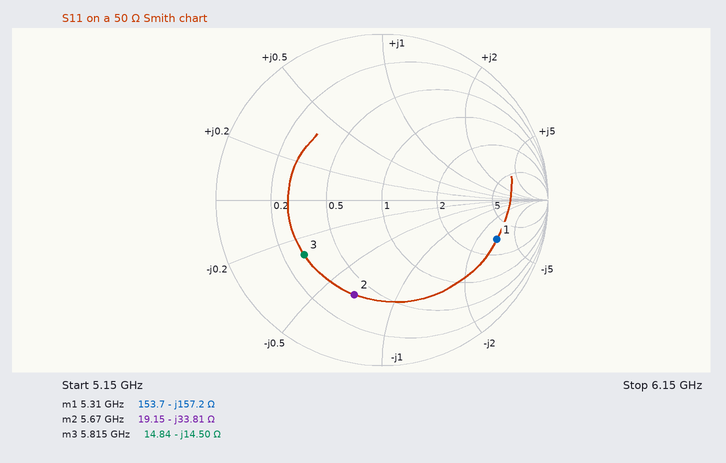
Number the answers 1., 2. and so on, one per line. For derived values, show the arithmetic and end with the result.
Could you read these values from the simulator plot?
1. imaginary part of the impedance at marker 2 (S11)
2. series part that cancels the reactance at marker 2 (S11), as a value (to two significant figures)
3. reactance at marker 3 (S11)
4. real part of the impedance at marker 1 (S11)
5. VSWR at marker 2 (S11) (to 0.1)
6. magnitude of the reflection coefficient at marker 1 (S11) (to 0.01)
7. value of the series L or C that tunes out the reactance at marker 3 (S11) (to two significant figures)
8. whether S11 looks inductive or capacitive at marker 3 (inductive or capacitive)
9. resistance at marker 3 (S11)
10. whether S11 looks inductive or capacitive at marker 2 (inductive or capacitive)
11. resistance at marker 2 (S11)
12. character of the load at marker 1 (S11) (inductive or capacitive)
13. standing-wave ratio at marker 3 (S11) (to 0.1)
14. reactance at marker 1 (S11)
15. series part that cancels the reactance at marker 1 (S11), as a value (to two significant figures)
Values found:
1. -33.81 Ω
2. L = 33.81 Ω/(2π × 5.67 GHz) ≈ 949 pH, so 950 pH to two significant figures
3. -14.50 Ω
4. 153.7 Ω
5. 3.9
6. 0.73
7. L = 14.5 Ω/(2π × 5.815 GHz) ≈ 397 pH, so 400 pH to two significant figures
8. capacitive
9. 14.84 Ω
10. capacitive
11. 19.15 Ω
12. capacitive
13. 3.7
14. -157.2 Ω
15. L = 157.2 Ω/(2π × 5.31 GHz) ≈ 4.7 nH
